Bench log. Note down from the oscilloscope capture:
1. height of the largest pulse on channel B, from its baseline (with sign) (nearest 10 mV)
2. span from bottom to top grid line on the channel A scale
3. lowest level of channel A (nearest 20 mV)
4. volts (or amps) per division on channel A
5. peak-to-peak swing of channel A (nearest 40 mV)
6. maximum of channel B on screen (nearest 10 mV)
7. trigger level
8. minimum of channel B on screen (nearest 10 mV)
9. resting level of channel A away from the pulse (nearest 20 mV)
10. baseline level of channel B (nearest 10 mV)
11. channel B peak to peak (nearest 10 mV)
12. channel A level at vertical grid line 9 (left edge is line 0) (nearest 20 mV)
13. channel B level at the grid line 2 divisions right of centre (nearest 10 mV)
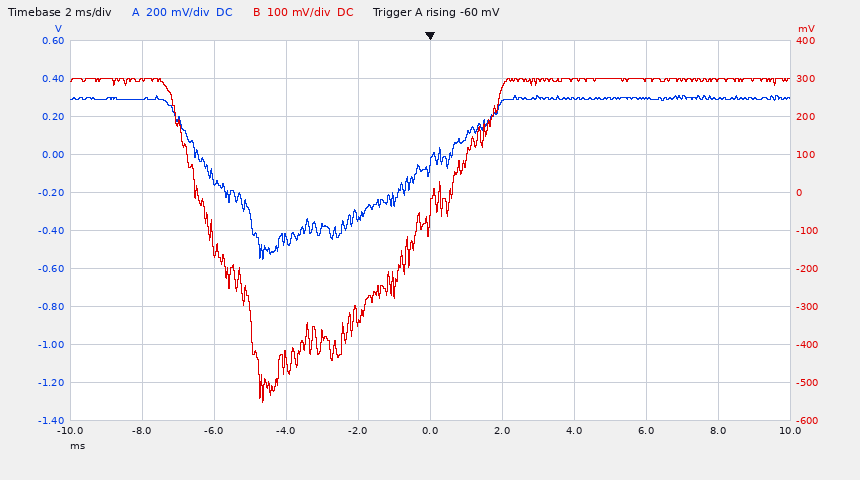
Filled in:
-850 mV
2 V
-560 mV
200 mV
880 mV
300 mV
-60 mV
-550 mV
300 mV
300 mV
850 mV
300 mV
300 mV
